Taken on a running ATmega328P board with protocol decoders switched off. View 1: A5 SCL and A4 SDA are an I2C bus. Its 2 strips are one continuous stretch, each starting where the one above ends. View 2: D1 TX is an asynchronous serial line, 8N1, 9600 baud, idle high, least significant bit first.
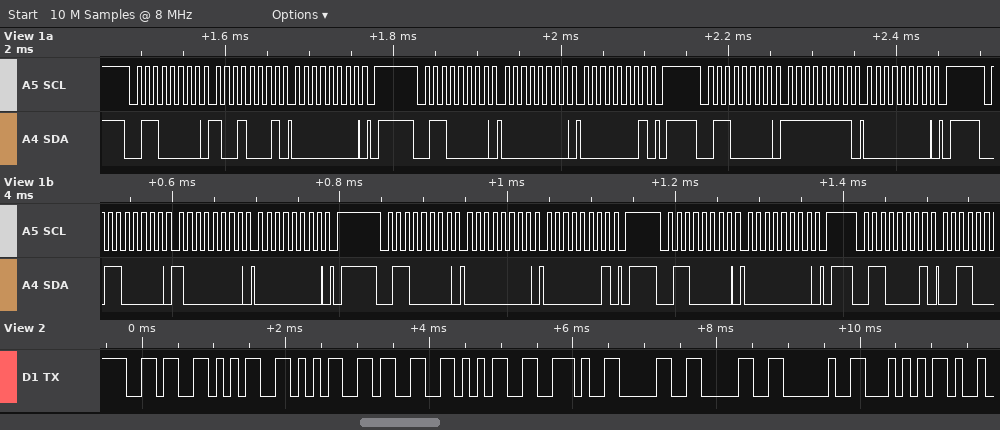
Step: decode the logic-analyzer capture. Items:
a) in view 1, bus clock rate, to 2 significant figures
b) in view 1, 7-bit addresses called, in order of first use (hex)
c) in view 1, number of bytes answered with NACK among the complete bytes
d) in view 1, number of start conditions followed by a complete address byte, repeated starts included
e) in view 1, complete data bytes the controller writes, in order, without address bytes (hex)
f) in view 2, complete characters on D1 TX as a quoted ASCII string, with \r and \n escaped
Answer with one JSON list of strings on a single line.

["100 kHz", "0x30", "0", "7", "91 00 00 01 FF 00 80 00 00 01 00", "\"65535.00 T\""]
